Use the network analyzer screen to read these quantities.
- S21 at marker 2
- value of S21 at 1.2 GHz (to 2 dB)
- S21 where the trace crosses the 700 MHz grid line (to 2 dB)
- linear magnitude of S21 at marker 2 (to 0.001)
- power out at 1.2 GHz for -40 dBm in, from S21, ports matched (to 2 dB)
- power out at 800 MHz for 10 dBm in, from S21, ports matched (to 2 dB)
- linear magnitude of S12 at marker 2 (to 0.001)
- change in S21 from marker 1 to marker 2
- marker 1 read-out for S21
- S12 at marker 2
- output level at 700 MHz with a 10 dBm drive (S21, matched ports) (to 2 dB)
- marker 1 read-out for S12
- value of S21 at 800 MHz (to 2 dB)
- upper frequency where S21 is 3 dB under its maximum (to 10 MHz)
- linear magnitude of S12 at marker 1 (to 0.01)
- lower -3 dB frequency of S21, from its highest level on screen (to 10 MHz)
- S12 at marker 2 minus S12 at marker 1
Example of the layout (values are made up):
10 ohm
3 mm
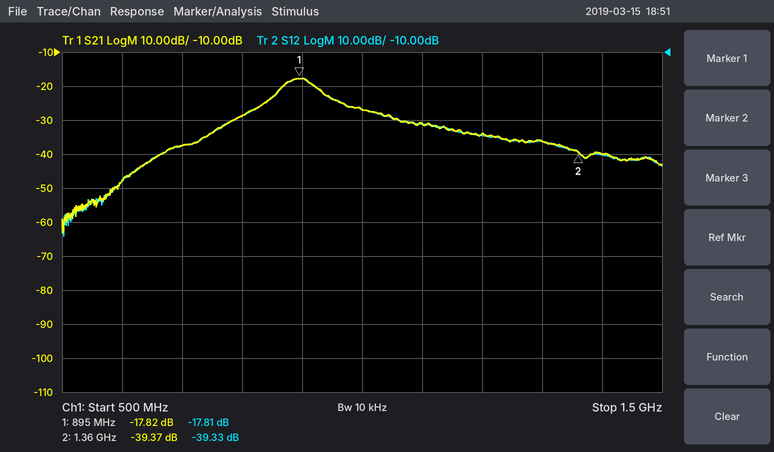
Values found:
-39.37 dB
-34 dB
-38 dB
0.011
-74 dBm
-18 dBm
0.011
-21.55 dB
-17.82 dB
-39.33 dB
-28 dBm
-17.81 dB
-28 dB
930 MHz
0.13
860 MHz
-21.52 dB
